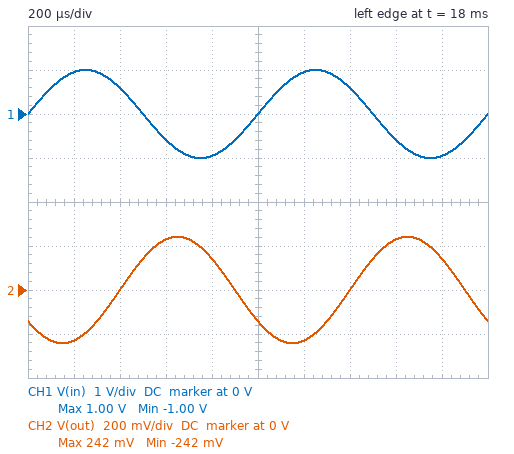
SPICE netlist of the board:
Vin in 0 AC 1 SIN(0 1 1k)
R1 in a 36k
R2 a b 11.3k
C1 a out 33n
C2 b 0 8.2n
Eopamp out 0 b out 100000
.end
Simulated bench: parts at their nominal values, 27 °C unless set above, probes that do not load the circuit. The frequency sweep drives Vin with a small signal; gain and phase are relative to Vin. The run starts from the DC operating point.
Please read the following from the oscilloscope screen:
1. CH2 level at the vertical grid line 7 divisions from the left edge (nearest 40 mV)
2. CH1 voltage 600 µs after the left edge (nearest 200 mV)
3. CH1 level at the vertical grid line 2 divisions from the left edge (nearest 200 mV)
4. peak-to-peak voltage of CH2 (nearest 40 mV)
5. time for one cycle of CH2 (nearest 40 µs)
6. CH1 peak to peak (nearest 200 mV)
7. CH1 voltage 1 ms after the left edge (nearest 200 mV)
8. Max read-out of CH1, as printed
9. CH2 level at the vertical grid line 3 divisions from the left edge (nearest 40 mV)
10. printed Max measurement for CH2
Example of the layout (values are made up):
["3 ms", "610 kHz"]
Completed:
["0 V", "-600 mV", "600 mV", "480 mV", "1.00 ms", "2.0 V", "0 V", "1.00 V", "240 mV", "242 mV"]
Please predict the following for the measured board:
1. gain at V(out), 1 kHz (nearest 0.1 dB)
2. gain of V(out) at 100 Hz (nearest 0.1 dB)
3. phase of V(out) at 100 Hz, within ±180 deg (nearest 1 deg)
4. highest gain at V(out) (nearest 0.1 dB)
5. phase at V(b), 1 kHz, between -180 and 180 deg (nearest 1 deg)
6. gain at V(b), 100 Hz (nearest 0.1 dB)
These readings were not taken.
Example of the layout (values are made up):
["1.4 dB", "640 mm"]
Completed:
["-12.3 dB", "0.1 dB", "-14 deg", "0.5 dB", "-144 deg", "0.1 dB"]
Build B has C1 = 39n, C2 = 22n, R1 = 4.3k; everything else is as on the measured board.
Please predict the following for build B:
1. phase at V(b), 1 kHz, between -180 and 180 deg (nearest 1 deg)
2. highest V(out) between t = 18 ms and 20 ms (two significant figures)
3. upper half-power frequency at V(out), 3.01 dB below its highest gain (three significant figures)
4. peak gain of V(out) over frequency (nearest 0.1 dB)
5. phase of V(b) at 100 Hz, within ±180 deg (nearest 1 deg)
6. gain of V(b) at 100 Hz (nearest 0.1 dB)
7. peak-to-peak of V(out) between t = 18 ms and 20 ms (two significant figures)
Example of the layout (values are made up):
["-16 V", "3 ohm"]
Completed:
["-107 deg", "440 mV", "638 Hz", "0 dB", "-12 deg", "-0.1 dB", "890 mV"]
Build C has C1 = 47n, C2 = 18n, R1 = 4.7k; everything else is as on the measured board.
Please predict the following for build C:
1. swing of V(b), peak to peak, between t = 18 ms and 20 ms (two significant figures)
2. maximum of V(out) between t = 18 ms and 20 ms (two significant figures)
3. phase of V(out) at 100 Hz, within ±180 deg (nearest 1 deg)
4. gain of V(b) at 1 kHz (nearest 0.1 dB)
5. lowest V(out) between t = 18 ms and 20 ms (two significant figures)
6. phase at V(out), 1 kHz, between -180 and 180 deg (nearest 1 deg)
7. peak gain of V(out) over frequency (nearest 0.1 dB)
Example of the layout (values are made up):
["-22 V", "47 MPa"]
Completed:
["1.0 V", "510 mV", "-10 deg", "-5.9 dB", "-510 mV", "-113 deg", "0 dB"]
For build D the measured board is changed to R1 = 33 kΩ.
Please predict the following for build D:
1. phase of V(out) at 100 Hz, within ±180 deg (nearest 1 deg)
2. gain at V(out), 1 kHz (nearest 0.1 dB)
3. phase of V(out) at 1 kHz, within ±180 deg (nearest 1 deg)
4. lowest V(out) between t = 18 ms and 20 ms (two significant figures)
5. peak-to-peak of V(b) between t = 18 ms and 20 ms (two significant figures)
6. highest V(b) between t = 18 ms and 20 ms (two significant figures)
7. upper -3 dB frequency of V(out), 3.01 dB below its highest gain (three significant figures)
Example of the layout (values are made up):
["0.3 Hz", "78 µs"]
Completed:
["-13 deg", "-11.5 dB", "-143 deg", "-270 mV", "530 mV", "270 mV", "568 Hz"]
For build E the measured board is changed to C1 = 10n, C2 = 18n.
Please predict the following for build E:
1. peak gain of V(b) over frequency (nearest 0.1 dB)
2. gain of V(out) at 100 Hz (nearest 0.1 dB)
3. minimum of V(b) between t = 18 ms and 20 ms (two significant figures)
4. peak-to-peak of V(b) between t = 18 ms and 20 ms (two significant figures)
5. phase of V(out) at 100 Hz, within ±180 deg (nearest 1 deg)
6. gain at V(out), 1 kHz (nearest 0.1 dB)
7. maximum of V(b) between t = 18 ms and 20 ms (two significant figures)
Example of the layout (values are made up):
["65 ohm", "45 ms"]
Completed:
["0 dB", "-0.9 dB", "-180 mV", "350 mV", "-29 deg", "-15.1 dB", "180 mV"]
